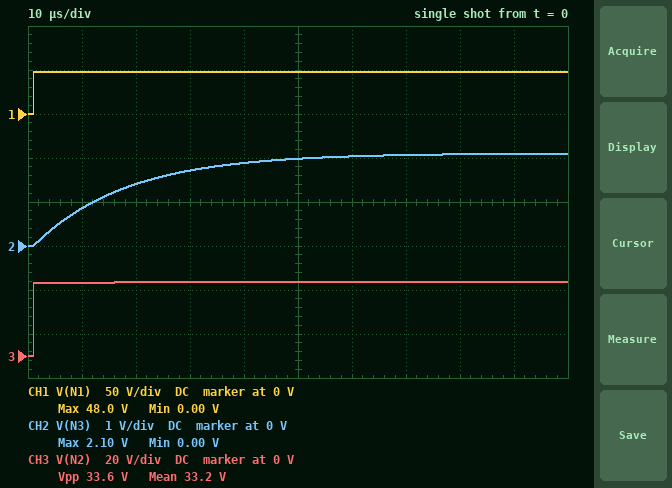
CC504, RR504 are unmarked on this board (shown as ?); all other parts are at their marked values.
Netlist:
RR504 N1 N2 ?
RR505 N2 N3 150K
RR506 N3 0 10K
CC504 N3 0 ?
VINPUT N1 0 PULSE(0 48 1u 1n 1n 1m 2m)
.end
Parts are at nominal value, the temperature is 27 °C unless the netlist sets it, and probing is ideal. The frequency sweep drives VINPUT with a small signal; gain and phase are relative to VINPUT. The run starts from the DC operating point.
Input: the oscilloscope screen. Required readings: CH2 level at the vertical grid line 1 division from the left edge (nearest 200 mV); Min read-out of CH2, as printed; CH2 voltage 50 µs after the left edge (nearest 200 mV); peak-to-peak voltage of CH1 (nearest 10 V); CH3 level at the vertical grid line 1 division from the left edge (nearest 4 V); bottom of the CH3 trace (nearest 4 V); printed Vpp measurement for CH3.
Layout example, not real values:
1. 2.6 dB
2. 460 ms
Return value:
1. 800 mV
2. 0.00 V
3. 2.0 V
4. 50 V
5. 32 V
6. 0 V
7. 33.6 V
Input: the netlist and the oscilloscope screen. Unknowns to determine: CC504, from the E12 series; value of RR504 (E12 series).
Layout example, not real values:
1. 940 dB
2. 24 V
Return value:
1. 1.8 nF
2. 68 kΩ
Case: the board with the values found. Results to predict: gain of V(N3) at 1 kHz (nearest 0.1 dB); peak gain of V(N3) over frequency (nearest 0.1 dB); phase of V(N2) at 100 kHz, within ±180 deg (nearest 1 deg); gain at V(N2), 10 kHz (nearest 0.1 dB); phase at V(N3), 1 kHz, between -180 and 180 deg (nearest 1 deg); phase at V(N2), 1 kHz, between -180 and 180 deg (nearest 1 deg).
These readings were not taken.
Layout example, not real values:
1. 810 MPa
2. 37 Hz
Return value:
1. -27.2 dB
2. -27.2 dB
3. 0 deg
4. -3.2 dB
5. -6 deg
6. 0 deg
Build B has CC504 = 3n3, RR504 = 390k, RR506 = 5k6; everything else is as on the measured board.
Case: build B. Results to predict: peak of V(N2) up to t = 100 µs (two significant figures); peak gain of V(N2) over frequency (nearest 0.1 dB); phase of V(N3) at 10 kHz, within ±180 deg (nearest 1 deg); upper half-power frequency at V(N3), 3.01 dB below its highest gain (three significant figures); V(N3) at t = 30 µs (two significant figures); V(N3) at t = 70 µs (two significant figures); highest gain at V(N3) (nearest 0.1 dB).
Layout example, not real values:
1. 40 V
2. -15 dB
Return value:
1. 14 V
2. -10.9 dB
3. -49 deg
4. 8.70 kHz
5. 390 mV
6. 480 mV
7. -39.8 dB
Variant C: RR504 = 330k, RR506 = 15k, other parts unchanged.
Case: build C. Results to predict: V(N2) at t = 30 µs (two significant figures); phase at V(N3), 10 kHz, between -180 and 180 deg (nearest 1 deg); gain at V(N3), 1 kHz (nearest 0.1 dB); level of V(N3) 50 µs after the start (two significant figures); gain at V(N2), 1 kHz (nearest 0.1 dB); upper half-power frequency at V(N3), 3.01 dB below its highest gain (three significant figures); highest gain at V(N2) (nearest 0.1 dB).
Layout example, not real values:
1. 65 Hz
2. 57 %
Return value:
1. 16 V
2. -59 deg
3. -30.5 dB
4. 1.2 V
5. -9.6 dB
6. 6.08 kHz
7. -9.5 dB
